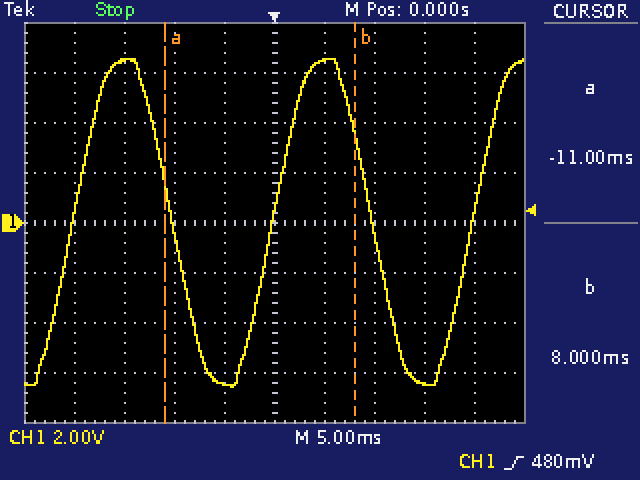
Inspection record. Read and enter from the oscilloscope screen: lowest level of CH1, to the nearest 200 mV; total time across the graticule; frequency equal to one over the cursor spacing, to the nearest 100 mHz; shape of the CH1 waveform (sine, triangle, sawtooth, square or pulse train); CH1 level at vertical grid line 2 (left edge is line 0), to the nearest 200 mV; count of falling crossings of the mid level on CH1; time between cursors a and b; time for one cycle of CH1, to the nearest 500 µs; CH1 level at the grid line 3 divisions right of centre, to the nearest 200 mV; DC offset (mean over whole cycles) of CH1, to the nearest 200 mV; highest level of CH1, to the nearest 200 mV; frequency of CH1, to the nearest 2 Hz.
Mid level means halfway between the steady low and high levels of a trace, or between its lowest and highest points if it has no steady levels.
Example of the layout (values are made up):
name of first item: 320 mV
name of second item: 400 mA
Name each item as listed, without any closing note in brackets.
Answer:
lowest level of CH1, to the nearest 200 mV: -6.6 V
total time across the graticule: 50 ms
frequency equal to one over the cursor spacing, to the nearest 100 mHz: 52.6 Hz
shape of the CH1 waveform: sine
CH1 level at vertical grid line 2 (left edge is line 0), to the nearest 200 mV: 6.4 V
count of falling crossings of the mid level on CH1: 2
time between cursors a and b: 19.0 ms
time for one cycle of CH1, to the nearest 500 µs: 20.0 ms
CH1 level at the grid line 3 divisions right of centre, to the nearest 200 mV: -6.4 V
DC offset (mean over whole cycles) of CH1, to the nearest 200 mV: 0.0 V
highest level of CH1, to the nearest 200 mV: 6.6 V
frequency of CH1, to the nearest 2 Hz: 50 Hz
